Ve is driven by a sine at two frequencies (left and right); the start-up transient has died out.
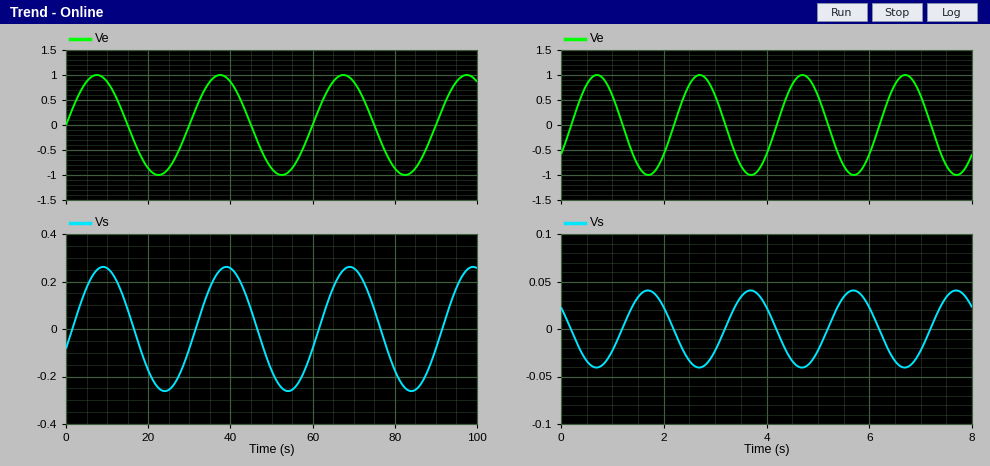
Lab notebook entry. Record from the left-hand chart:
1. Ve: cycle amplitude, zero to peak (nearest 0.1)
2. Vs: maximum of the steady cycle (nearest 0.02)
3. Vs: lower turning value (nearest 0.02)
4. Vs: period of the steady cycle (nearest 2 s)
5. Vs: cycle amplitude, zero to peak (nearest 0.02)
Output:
1.0
0.26
-0.26
30 s
0.26
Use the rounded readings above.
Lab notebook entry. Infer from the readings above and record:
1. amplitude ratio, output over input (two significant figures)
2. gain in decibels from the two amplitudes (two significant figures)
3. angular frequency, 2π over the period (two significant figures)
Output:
0.26
-12 dB
0.21 rad/s
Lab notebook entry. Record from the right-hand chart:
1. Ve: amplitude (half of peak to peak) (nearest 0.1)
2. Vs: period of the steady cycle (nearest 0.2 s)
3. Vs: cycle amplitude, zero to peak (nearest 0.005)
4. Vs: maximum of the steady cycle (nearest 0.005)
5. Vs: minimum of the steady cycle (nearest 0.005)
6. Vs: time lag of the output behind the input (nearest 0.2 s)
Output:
1.0
2.0 s
0.040
0.040
-0.040
1.0 s
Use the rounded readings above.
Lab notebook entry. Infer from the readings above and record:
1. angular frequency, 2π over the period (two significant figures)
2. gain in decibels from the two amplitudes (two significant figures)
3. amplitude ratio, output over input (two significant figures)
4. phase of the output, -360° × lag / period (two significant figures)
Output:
3.1 rad/s
-28 dB
0.040
-180°
